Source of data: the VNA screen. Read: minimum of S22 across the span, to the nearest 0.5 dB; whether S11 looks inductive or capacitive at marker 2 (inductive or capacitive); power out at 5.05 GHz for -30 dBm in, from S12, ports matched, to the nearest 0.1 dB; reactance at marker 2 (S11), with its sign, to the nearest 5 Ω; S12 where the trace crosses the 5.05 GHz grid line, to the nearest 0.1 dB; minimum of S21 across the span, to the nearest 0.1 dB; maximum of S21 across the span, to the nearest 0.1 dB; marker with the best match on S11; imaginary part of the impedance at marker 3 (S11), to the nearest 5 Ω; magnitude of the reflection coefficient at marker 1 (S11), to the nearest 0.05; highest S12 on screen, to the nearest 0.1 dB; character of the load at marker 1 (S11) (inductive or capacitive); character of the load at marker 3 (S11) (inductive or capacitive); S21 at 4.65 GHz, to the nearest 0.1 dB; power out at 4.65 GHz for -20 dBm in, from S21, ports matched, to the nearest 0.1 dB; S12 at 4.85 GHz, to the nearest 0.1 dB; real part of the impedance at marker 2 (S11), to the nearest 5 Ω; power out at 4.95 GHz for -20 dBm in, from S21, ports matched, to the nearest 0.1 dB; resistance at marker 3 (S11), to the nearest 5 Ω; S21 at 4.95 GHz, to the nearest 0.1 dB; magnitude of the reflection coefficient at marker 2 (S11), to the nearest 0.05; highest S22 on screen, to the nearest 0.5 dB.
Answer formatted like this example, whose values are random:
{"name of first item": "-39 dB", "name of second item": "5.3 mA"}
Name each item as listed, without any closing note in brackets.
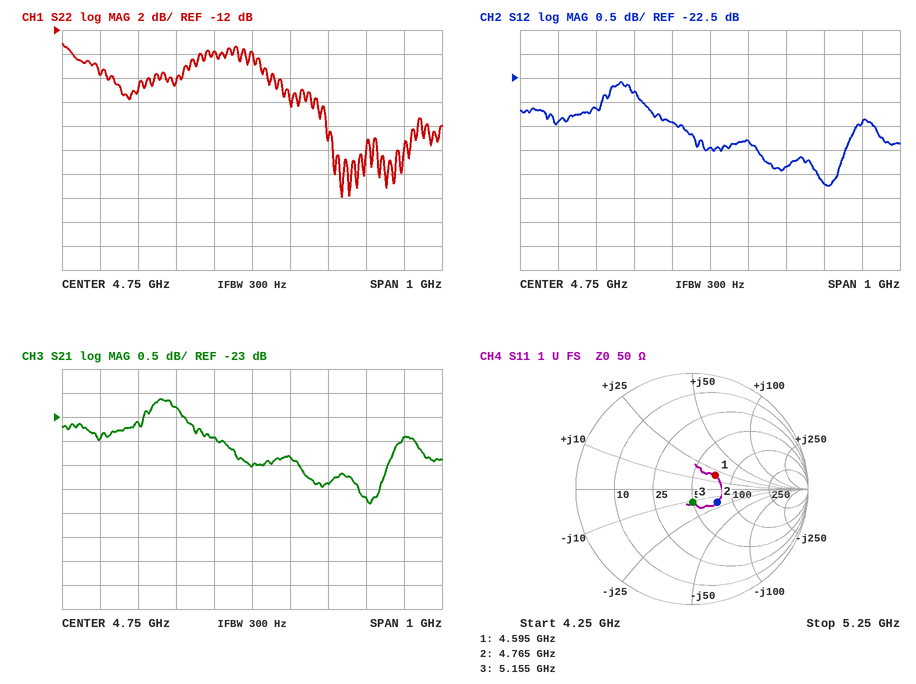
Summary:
{"minimum of S22 across the span, to the nearest 0.5 dB": "-26.0 dB", "whether S11 looks inductive or capacitive at marker 2": "capacitive", "power out at 5.05 GHz for -30 dBm in, from S12, ports matched, to the nearest 0.1 dB": "-54.7 dBm", "reactance at marker 2 (S11), with its sign, to the nearest 5 Ω": "-20 Ω", "S12 where the trace crosses the 5.05 GHz grid line, to the nearest 0.1 dB": "-24.7 dB", "minimum of S21 across the span, to the nearest 0.1 dB": "-24.8 dB", "maximum of S21 across the span, to the nearest 0.1 dB": "-22.6 dB", "marker with the best match on S11": "marker 3", "imaginary part of the impedance at marker 3 (S11), to the nearest 5 Ω": "-10 Ω", "magnitude of the reflection coefficient at marker 1 (S11), to the nearest 0.05": "0.25", "highest S12 on screen, to the nearest 0.1 dB": "-22.6 dB", "character of the load at marker 1 (S11)": "inductive", "character of the load at marker 3 (S11)": "capacitive", "S21 at 4.65 GHz, to the nearest 0.1 dB": "-23.4 dB", "power out at 4.65 GHz for -20 dBm in, from S21, ports matched, to the nearest 0.1 dB": "-43.4 dBm", "S12 at 4.85 GHz, to the nearest 0.1 dB": "-23.8 dB", "real part of the impedance at marker 2 (S11), to the nearest 5 Ω": "75 Ω", "power out at 4.95 GHz for -20 dBm in, from S21, ports matched, to the nearest 0.1 dB": "-44.4 dBm", "resistance at marker 3 (S11), to the nearest 5 Ω": "50 Ω", "S21 at 4.95 GHz, to the nearest 0.1 dB": "-24.4 dB", "magnitude of the reflection coefficient at marker 2 (S11), to the nearest 0.05": "0.25", "highest S22 on screen, to the nearest 0.5 dB": "-13.0 dB"}
